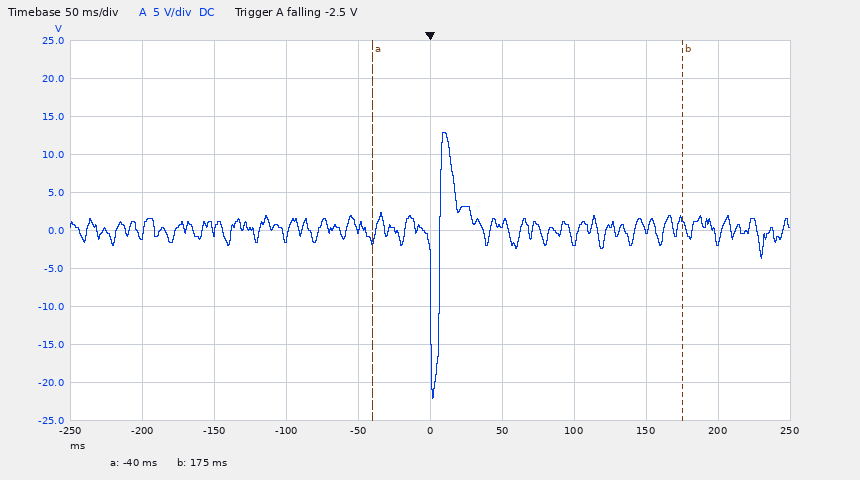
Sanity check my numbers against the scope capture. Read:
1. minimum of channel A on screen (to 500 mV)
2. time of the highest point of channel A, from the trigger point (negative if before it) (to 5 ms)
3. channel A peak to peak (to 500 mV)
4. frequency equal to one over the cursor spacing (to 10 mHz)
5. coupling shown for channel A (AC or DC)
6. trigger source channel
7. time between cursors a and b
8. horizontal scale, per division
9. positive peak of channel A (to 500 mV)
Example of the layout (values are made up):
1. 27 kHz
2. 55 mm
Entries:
1. -22.0 V
2. +10 ms
3. 35.0 V
4. 4.65 Hz
5. DC
6. channel A
7. 215 ms
8. 50 ms
9. 13.0 V
